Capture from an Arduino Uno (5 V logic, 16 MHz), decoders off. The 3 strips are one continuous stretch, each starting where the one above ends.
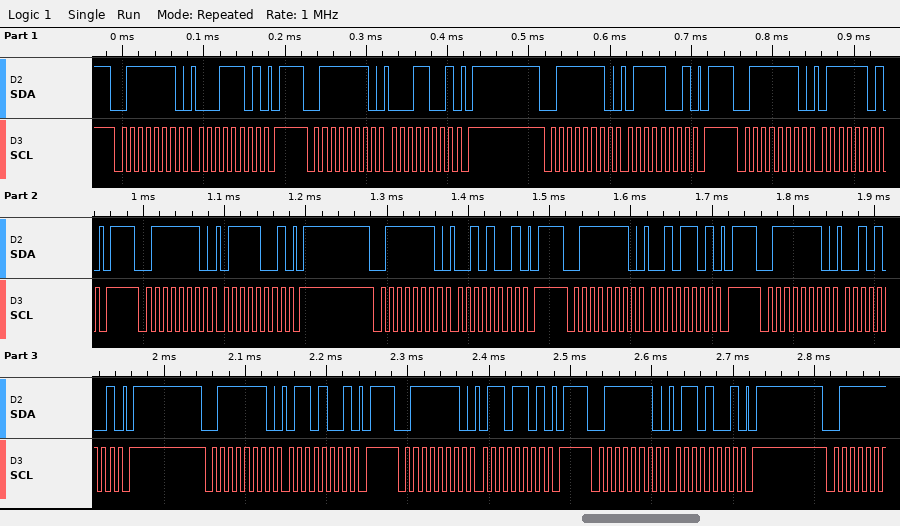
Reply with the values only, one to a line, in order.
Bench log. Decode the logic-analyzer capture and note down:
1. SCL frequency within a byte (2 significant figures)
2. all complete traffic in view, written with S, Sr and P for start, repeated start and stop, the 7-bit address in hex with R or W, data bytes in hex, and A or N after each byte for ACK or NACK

100 kHz
S 3FW A 1D A P S 3FW A 19 A P S 3FW A 79 A P S 3FW A 7D A P S 3FW A 79 A P S 3FW A 29 A P S 3FW A 2D A P S 3FW A 29 A P S 3FW A 69 A P S 3FW A 6D A P S 3FW A 69 A P
